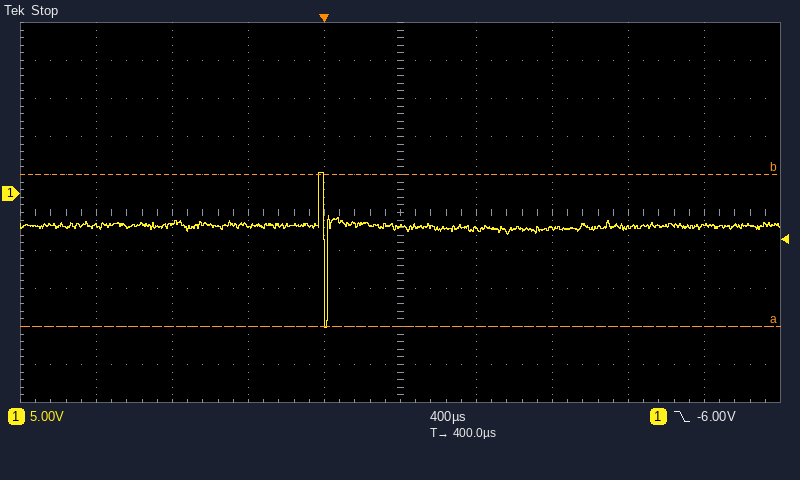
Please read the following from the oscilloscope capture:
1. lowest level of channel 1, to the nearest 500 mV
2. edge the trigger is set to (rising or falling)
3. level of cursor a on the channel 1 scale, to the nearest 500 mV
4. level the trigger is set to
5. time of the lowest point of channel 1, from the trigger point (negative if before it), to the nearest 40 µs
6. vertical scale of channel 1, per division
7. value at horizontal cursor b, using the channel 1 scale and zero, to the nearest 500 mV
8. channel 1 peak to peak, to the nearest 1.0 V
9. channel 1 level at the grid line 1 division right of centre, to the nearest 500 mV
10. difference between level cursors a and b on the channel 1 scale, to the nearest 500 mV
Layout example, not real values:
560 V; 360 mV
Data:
-17.5 V; falling; -17.5 V; -6.00 V; 0 µs; 5 V; 2.5 V; 20.0 V; -4.5 V; 20.0 V
